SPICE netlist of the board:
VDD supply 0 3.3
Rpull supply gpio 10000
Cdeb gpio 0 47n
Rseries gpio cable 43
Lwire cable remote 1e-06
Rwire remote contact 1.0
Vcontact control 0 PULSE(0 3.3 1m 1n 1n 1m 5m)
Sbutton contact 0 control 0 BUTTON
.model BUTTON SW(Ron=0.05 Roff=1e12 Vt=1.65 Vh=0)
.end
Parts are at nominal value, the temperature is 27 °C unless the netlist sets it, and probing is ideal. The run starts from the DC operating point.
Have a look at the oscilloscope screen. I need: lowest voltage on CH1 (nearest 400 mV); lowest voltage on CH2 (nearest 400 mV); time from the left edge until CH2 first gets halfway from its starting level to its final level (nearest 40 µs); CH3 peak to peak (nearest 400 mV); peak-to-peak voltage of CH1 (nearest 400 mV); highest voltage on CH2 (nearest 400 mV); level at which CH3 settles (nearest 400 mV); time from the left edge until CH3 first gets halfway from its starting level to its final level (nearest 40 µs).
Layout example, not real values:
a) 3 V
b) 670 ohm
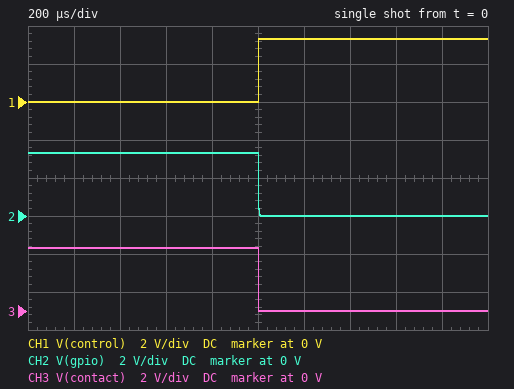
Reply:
a) 0 V
b) 0 V
c) 1.00 ms
d) 3.2 V
e) 3.2 V
f) 3.2 V
g) 0 V
h) 1.00 ms
